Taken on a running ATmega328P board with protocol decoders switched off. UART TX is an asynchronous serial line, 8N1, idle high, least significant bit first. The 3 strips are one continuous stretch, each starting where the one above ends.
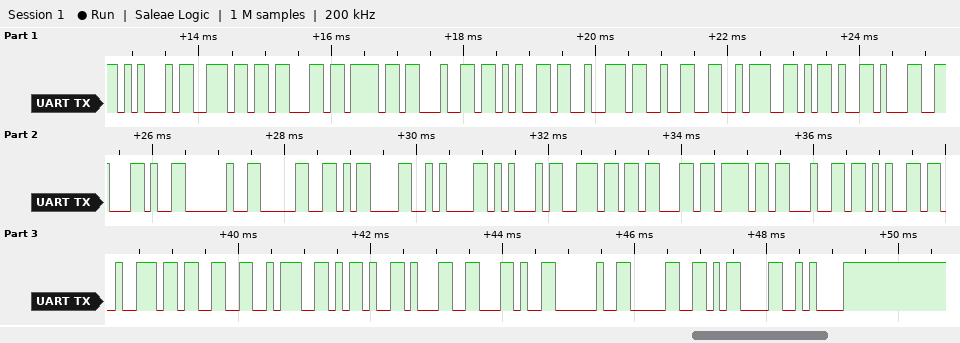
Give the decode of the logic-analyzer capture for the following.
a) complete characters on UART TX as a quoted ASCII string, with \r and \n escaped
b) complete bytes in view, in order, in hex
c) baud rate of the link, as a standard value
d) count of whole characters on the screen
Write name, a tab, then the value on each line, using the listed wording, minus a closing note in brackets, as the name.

complete characters on UART TX as a quoted ASCII string, with \r and \n escaped	"Encoder2:-1, 0\r\nEncoder3:-1, 0\r\n"
complete bytes in view, in order, in hex	0x45 0x6E 0x63 0x6F 0x64 0x65 0x72 0x32 0x3A 0x2D 0x31 0x2C 0x20 0x30 0x0D 0x0A 0x45 0x6E 0x63 0x6F 0x64 0x65 0x72 0x33 0x3A 0x2D 0x31 0x2C 0x20 0x30 0x0D 0x0A
baud rate of the link, as a standard value	9600 baud
count of whole characters on the screen	32
